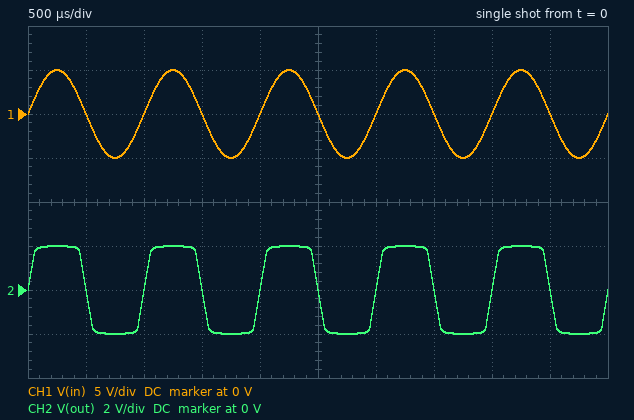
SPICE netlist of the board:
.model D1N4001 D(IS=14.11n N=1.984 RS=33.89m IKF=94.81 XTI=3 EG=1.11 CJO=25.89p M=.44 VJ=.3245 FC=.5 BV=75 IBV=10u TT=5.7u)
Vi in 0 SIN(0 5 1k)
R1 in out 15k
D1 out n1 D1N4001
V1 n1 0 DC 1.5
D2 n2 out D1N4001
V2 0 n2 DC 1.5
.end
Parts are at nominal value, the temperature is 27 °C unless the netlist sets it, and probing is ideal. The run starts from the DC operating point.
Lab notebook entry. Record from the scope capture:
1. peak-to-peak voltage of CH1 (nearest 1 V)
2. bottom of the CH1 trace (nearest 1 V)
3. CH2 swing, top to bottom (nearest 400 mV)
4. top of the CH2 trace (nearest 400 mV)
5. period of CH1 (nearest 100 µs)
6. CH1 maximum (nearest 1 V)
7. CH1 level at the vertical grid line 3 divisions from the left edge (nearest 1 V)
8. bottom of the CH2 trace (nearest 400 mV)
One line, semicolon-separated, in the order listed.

10 V; -5 V; 4.0 V; 2.0 V; 1.0 ms; 5 V; 0 V; -2.0 V
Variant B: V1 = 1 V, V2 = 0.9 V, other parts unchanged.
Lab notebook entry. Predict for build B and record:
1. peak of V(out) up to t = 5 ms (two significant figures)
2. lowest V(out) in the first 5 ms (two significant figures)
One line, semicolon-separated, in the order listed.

1.5 V; -1.4 V
